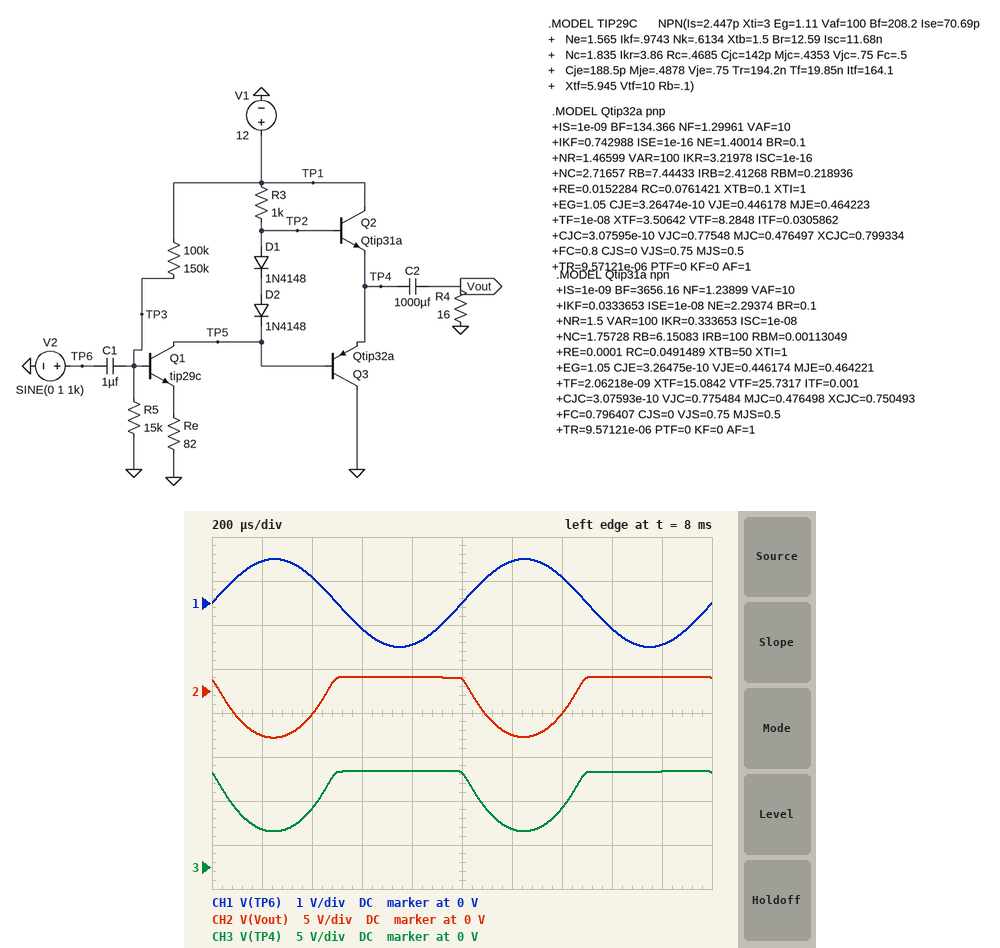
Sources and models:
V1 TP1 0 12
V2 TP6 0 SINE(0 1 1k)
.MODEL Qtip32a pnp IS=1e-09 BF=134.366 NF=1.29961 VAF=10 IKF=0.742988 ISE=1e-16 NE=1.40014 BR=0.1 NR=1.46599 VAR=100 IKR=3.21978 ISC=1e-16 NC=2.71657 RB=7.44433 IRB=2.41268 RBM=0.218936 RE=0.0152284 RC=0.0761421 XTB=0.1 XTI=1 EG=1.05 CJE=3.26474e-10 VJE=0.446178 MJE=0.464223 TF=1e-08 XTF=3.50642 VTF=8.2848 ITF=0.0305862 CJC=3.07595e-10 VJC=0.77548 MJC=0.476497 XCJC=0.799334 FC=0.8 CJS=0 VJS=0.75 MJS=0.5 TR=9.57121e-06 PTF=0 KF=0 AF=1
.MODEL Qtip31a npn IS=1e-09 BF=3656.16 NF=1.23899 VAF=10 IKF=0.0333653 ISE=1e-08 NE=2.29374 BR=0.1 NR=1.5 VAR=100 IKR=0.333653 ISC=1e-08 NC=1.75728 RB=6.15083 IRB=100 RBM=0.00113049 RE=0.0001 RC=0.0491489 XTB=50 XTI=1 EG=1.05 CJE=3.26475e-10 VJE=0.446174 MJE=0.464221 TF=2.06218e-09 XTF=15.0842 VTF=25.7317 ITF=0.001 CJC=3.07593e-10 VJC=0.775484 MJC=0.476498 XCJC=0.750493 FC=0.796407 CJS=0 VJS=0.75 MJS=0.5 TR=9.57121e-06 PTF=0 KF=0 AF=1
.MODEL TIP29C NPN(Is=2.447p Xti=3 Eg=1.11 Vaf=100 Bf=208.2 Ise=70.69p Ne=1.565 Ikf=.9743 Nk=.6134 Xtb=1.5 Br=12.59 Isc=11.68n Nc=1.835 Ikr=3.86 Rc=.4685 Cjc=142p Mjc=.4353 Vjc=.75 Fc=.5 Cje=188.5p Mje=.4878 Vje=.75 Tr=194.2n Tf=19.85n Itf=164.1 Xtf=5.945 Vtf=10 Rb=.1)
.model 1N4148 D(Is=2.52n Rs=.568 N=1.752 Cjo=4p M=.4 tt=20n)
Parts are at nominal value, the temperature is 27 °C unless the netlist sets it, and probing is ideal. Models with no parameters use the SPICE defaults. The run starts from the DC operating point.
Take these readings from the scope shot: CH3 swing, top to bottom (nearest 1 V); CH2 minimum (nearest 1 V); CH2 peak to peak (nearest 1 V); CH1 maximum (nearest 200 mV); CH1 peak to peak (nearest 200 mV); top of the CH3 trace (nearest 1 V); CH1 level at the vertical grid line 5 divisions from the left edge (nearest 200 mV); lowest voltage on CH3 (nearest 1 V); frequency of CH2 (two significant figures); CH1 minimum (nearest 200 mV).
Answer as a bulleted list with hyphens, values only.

- 7 V
- -5 V
- 7 V
- 1.0 V
- 2.0 V
- 11 V
- 0 V
- 4 V
- 1.0 kHz
- -1.0 V
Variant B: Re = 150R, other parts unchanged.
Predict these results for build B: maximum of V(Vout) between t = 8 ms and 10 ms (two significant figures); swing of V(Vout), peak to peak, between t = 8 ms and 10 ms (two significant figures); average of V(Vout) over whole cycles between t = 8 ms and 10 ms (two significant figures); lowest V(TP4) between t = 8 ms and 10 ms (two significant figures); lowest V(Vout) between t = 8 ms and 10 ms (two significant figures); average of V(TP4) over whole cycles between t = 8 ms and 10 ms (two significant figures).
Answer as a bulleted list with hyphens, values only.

- 1.2 V
- 4.8 V
- -460 mV
- 6.2 V
- -3.6 V
- 9.3 V
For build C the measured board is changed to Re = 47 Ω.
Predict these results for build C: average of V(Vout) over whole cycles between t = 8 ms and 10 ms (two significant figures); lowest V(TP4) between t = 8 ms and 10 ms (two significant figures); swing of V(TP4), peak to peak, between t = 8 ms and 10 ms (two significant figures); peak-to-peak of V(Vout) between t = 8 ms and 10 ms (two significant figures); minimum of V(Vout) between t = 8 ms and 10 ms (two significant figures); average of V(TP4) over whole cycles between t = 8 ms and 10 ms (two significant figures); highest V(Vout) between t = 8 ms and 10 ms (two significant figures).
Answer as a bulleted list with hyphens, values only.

- -840 mV
- 2.1 V
- 8.7 V
- 8.8 V
- -7.0 V
- 8.2 V
- 1.8 V
